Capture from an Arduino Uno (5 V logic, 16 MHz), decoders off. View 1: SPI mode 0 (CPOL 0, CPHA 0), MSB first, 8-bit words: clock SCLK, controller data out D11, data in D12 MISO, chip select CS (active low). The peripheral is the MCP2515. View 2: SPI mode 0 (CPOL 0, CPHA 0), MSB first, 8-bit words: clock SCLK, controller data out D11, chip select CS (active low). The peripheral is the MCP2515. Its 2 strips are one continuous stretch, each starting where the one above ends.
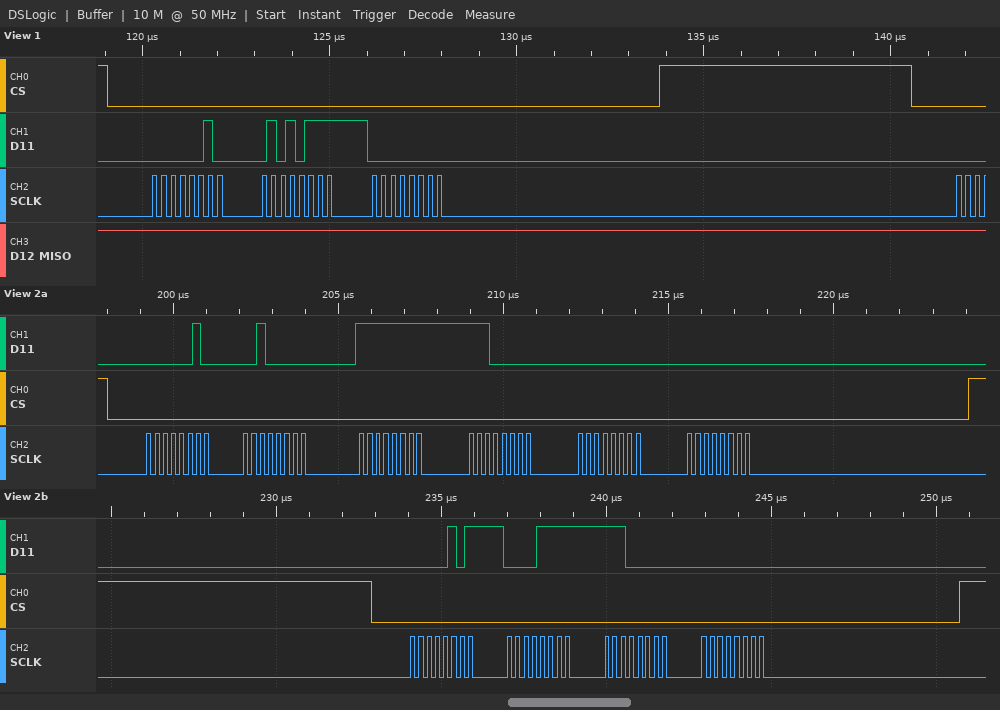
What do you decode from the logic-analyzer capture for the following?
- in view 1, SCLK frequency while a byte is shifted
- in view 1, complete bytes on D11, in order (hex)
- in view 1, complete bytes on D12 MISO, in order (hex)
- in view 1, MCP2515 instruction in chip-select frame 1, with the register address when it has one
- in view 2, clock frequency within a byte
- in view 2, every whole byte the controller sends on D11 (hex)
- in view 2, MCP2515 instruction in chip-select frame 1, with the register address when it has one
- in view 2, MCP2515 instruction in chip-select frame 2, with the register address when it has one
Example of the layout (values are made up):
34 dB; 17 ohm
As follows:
4 MHz; 0x02 0x57 0x00; 0xFF 0xFF 0xFF; WRITE 0x57; 4 MHz; 02 20 FF E0 00 00 05 0F E0 00; WRITE 0x20; BIT MODIFY 0x0F
